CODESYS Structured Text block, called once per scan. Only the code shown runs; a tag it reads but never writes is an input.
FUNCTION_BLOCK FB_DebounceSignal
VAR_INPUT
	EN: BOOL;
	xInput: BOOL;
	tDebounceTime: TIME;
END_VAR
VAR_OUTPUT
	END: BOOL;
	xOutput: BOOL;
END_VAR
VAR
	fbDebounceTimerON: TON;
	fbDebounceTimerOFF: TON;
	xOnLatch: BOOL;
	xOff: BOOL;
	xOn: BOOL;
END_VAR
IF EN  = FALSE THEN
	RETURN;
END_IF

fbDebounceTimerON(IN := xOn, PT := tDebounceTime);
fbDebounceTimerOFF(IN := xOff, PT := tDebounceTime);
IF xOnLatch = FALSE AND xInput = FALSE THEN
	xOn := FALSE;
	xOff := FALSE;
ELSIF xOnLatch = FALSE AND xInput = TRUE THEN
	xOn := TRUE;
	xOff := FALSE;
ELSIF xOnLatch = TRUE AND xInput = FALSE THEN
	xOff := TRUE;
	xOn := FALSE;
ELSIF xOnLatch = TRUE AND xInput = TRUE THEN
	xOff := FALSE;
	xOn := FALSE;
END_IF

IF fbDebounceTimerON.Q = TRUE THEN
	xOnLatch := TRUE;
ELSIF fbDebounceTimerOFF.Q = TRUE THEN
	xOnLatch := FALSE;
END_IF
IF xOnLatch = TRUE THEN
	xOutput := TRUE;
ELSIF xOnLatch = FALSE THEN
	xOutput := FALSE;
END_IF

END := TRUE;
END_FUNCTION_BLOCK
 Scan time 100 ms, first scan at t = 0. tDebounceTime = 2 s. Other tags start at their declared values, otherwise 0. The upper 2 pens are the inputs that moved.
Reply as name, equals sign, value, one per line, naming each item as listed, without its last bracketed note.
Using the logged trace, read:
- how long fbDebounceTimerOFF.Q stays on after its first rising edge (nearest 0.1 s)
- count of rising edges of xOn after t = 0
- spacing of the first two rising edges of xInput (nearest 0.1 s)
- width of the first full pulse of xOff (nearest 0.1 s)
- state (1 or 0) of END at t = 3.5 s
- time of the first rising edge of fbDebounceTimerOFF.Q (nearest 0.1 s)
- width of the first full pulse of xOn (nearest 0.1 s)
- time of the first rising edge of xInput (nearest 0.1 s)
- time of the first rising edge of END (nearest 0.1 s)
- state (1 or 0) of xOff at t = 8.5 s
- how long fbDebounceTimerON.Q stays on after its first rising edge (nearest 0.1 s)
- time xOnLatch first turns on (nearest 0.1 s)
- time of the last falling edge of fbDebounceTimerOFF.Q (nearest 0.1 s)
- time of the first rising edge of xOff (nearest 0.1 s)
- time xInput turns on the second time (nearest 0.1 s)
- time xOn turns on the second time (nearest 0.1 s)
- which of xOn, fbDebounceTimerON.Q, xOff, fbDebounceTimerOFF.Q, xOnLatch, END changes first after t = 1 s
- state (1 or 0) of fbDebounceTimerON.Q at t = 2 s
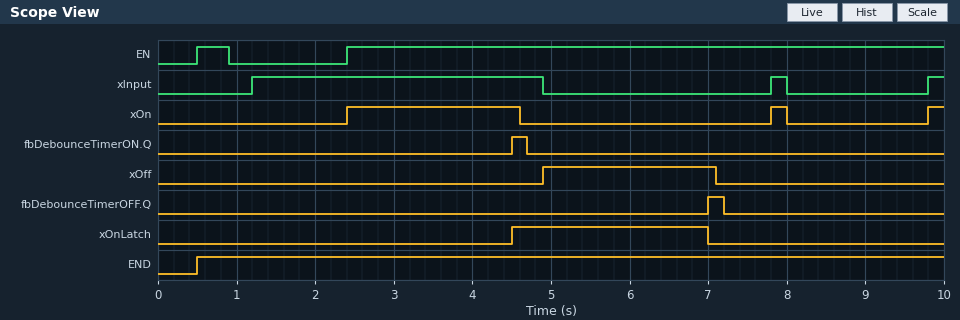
how long fbDebounceTimerOFF.Q stays on after its first rising edge = 0.2 s
count of rising edges of xOn after t = 0 = 3
spacing of the first two rising edges of xInput = 6.6 s
width of the first full pulse of xOff = 2.2 s
state (1 or 0) of END at t = 3.5 s = 1
time of the first rising edge of fbDebounceTimerOFF.Q = 7.0 s
width of the first full pulse of xOn = 2.2 s
time of the first rising edge of xInput = 1.2 s
time of the first rising edge of END = 0.5 s
state (1 or 0) of xOff at t = 8.5 s = 0
how long fbDebounceTimerON.Q stays on after its first rising edge = 0.2 s
time xOnLatch first turns on = 4.5 s
time of the last falling edge of fbDebounceTimerOFF.Q = 7.2 s
time of the first rising edge of xOff = 4.9 s
time xInput turns on the second time = 7.8 s
time xOn turns on the second time = 7.8 s
which of xOn, fbDebounceTimerON.Q, xOff, fbDebounceTimerOFF.Q, xOnLatch, END changes first after t = 1 s = xOn
state (1 or 0) of fbDebounceTimerON.Q at t = 2 s = 0
